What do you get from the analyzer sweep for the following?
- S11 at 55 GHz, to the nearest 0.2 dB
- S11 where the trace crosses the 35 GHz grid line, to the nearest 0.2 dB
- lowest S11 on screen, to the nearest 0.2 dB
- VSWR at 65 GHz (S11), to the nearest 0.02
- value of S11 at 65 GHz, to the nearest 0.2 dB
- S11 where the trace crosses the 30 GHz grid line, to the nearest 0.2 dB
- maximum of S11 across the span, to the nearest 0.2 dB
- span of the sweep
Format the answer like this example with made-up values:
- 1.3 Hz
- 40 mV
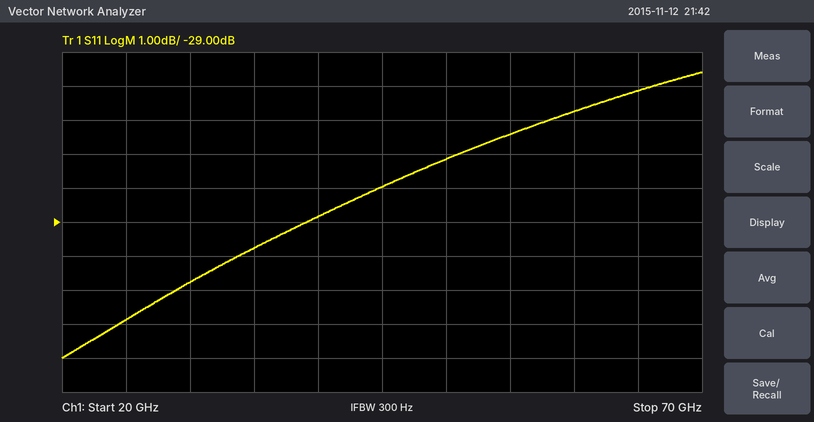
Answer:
- -26.4 dB
- -29.8 dB
- -33.0 dB
- 1.12
- -25.2 dB
- -30.8 dB
- -24.6 dB
- 50 GHz
